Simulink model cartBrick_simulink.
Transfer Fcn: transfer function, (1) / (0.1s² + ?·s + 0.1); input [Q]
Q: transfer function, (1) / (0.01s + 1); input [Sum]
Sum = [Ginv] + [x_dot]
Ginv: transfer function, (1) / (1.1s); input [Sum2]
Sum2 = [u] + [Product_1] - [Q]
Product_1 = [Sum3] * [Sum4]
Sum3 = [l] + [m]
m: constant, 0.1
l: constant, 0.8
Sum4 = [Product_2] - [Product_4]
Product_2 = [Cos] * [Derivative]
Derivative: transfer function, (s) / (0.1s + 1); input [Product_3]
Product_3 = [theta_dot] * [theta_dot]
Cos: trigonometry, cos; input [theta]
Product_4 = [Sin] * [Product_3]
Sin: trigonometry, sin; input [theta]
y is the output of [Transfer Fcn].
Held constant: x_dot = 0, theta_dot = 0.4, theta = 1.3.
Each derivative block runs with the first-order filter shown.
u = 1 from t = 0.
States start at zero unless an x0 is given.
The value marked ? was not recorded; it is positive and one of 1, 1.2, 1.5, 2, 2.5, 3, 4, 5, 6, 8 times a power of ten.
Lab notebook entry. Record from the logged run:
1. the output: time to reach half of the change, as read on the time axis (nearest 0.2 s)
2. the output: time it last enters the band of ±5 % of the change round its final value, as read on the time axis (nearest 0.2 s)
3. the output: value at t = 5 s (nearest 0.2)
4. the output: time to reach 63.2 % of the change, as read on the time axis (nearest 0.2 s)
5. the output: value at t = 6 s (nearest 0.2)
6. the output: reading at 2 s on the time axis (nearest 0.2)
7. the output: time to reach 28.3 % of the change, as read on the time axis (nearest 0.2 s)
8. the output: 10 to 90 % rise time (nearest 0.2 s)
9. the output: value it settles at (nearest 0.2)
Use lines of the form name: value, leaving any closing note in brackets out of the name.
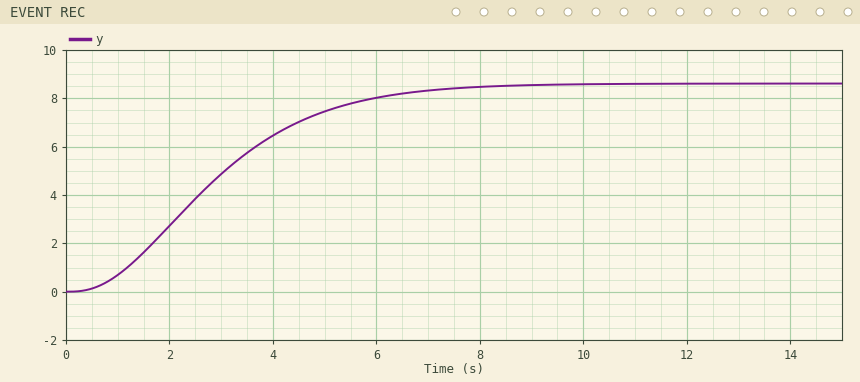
the output: time to reach half of the change, as read on the time axis: 2.8 s
the output: time it last enters the band of ±5 % of the change round its final value, as read on the time axis: 6.4 s
the output: value at t = 5 s: 7.4
the output: time to reach 63.2 % of the change, as read on the time axis: 3.4 s
the output: value at t = 6 s: 8.0
the output: reading at 2 s on the time axis: 2.8
the output: time to reach 28.3 % of the change, as read on the time axis: 1.8 s
the output: 10 to 90 % rise time: 4.4 s
the output: value it settles at: 8.6
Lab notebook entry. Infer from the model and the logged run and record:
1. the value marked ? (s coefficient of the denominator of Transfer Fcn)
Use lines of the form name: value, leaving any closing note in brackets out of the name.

the value marked ?: 0.2
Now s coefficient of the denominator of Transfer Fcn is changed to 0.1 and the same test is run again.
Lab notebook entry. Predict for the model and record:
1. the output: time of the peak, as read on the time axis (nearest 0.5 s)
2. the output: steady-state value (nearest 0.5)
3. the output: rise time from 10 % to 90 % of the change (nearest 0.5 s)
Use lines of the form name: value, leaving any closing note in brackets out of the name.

the output: time of the peak, as read on the time axis: 5.0 s
the output: steady-state value: 8.5
the output: rise time from 10 % to 90 % of the change: 2.5 s
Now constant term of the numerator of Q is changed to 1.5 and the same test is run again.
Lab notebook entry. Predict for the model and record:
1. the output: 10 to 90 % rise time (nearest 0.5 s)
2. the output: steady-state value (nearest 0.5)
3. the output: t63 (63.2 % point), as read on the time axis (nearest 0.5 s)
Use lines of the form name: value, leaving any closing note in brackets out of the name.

the output: 10 to 90 % rise time: 4.0 s
the output: steady-state value: 8.5
the output: t63 (63.2 % point), as read on the time axis: 3.0 s
